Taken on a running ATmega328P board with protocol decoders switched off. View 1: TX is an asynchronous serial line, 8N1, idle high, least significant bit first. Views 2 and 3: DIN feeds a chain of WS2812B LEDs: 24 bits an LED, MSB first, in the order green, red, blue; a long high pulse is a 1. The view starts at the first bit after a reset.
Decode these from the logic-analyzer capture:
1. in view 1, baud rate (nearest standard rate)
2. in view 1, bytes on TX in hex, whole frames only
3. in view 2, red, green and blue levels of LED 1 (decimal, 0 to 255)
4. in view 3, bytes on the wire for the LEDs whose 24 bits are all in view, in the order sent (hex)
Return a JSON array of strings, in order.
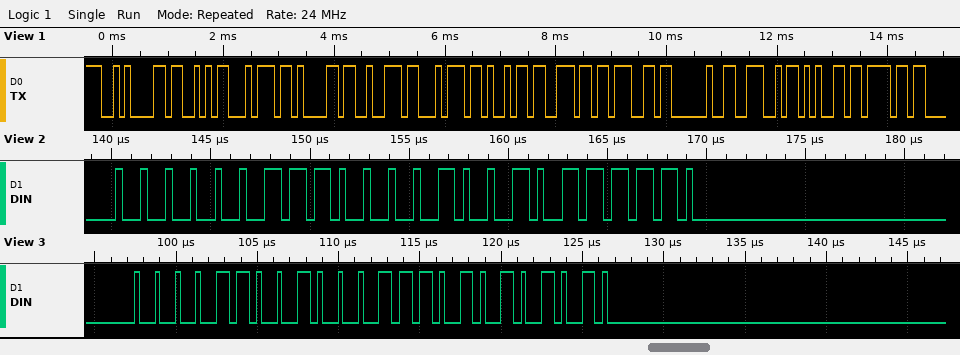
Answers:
["9600 baud", "0A 53 74 61 72 74 69 6E 67 20 4E 65 6F", "132, 3, 190", "0C 8E AA"]
